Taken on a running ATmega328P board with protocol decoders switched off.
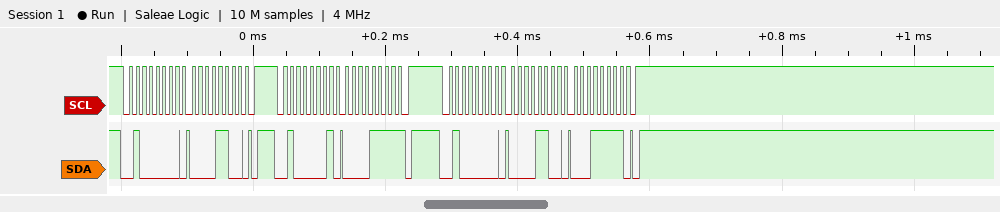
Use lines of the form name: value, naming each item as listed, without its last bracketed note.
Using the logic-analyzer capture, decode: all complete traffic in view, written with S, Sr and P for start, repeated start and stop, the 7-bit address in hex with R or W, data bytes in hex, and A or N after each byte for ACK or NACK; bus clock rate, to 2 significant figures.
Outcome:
all complete traffic in view, written with S, Sr and P for start, repeated start and stop, the 7-bit address in hex with R or W, data bytes in hex, and A or N after each byte for ACK or NACK: S 20W A 0C A P S 20R A 0F N P S 20W A 0C A 1F A P
bus clock rate, to 2 significant figures: 100 kHz
